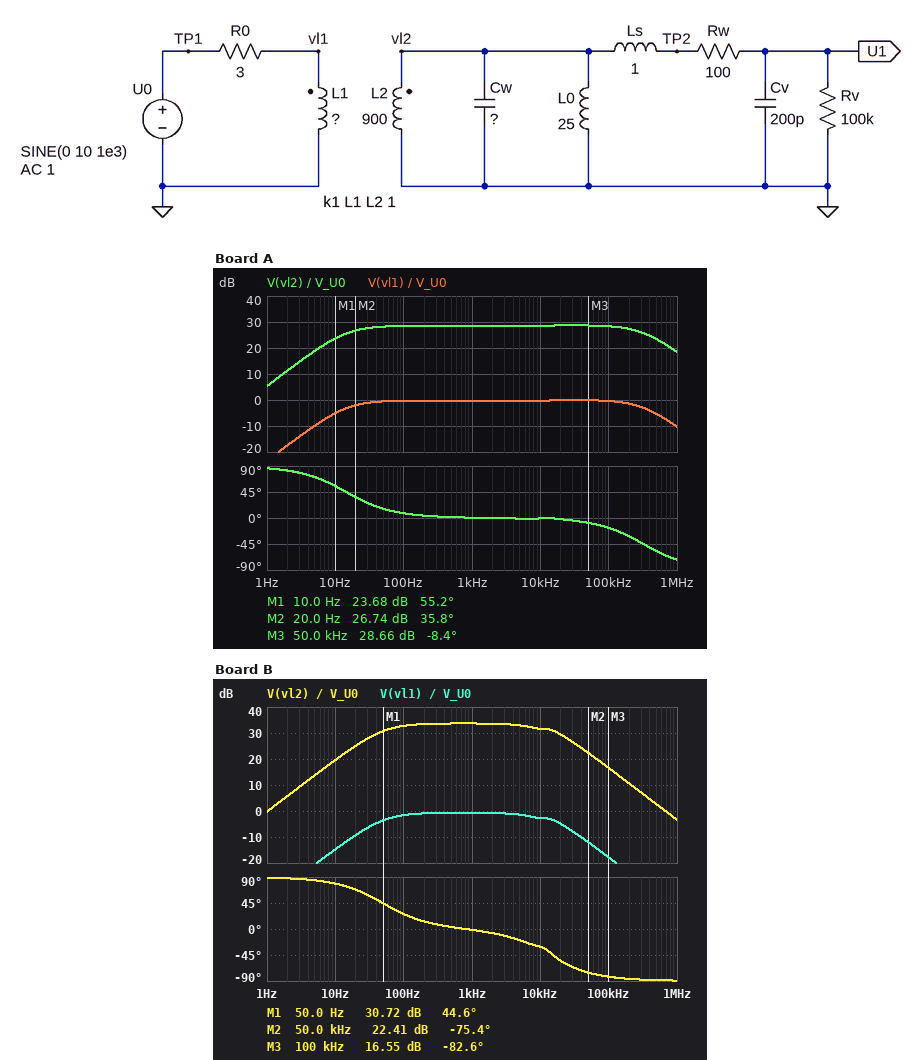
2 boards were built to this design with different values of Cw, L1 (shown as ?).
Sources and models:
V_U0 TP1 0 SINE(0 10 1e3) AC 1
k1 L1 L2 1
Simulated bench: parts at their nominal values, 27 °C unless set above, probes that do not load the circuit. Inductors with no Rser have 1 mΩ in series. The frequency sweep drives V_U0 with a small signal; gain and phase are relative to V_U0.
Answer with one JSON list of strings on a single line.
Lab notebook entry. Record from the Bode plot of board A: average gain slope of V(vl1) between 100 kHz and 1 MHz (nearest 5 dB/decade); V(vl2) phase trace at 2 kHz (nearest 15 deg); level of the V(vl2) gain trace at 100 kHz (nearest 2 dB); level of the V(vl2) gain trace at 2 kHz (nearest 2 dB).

["-10 dB/decade", "0 deg", "28 dB", "28 dB"]
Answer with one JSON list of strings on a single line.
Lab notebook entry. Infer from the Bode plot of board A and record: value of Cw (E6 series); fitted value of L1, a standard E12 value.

["220 pF", "1.2 H"]
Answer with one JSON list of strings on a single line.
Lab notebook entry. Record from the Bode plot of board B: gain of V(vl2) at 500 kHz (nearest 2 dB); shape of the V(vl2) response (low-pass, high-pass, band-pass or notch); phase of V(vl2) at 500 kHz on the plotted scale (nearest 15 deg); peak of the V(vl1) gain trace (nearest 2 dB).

["2 dB", "band-pass", "-90 deg", "0 dB"]
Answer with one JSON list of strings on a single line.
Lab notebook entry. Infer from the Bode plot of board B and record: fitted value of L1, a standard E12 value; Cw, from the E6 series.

["330 mH", "1.5 nF"]
